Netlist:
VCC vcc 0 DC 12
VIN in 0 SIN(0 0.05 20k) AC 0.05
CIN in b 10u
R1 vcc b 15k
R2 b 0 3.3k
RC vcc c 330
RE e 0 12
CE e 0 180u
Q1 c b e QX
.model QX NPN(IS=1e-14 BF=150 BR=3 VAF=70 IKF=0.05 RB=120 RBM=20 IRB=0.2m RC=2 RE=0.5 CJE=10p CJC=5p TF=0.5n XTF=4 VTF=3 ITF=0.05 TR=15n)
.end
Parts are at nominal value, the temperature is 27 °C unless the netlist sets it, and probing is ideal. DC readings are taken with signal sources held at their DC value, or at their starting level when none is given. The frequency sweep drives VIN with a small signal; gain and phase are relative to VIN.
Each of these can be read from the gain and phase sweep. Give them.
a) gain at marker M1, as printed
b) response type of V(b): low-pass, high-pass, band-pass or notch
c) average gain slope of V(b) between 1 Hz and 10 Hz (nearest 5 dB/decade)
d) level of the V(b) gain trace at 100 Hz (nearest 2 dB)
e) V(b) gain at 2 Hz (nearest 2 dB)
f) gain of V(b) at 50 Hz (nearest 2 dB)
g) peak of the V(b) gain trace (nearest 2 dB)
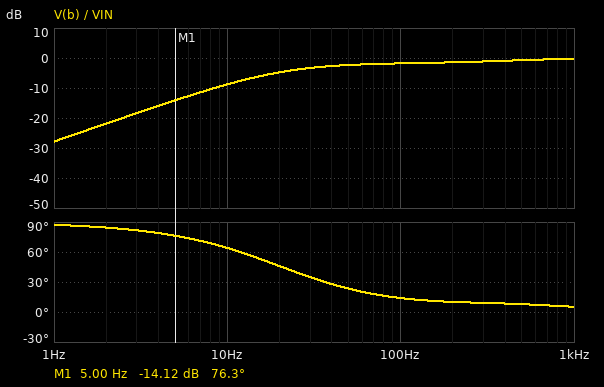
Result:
-14.12 dB
high-pass
20 dB/decade
-2 dB
-22 dB
-2 dB
0 dB
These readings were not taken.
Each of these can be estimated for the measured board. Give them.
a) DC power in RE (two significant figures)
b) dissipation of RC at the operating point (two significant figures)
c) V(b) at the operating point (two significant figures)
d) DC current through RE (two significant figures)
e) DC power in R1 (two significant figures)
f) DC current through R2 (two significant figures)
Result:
13 mW
350 mW
1.2 V
33 mA
7.8 mW
360 µA
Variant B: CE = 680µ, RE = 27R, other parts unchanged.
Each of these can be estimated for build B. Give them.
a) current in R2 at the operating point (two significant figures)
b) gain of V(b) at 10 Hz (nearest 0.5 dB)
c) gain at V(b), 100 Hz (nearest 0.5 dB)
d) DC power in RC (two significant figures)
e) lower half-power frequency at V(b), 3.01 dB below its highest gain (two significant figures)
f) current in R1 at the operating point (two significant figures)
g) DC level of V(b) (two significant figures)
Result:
450 µA
-7.0 dB
-3.0 dB
220 mW
110 Hz
700 µA
1.5 V
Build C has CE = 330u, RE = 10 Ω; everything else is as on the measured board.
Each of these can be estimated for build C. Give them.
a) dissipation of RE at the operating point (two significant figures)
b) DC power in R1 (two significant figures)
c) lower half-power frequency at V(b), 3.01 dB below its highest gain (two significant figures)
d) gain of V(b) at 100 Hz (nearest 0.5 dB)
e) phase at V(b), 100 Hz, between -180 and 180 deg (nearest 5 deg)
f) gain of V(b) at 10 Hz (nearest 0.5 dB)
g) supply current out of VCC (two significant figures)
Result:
12 mW
7.9 mW
73 Hz
-2.5 dB
20 deg
-10.0 dB
34 mA
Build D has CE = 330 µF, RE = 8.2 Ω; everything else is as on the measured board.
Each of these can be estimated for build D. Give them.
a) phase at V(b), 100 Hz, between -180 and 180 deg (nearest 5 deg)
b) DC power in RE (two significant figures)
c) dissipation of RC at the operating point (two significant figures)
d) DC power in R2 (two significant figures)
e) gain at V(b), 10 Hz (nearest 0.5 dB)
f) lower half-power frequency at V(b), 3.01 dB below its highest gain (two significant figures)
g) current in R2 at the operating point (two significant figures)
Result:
35 deg
10 mW
390 mW
360 µW
-18.0 dB
220 Hz
330 µA
